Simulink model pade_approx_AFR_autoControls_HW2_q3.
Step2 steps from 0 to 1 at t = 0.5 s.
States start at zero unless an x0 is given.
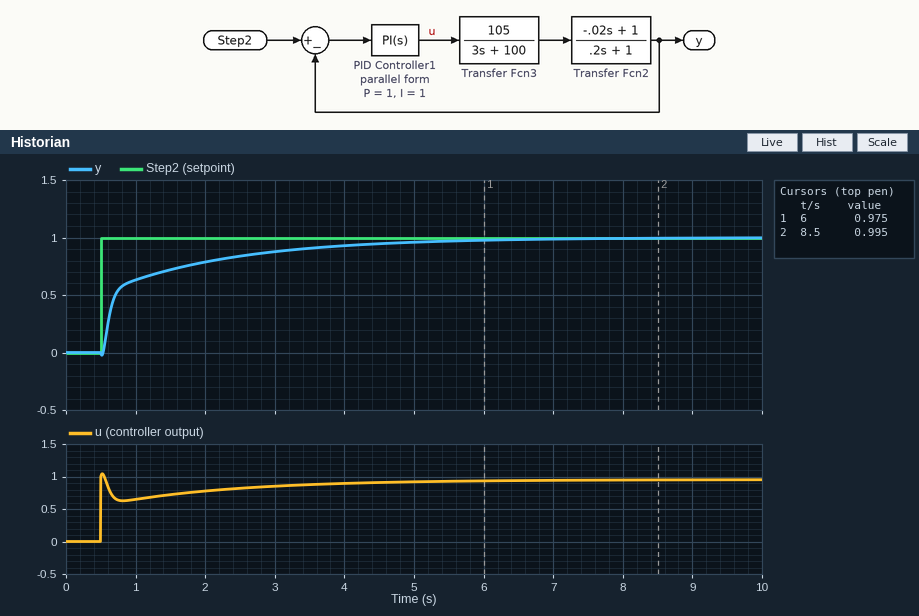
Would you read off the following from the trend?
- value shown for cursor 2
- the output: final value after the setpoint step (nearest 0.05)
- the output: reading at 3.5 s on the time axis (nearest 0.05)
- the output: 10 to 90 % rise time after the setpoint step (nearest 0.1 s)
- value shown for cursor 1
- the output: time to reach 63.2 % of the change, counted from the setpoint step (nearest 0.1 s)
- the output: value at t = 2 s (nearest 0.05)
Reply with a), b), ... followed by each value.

a) 0.995
b) 1.00
c) 0.90
d) 2.8 s
e) 0.975
f) 0.5 s
g) 0.80
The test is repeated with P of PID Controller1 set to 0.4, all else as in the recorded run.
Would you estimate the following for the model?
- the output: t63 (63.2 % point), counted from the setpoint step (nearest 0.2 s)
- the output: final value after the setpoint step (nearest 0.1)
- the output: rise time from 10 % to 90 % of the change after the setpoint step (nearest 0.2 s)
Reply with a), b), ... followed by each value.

a) 0.8 s
b) 1.0
c) 2.2 s
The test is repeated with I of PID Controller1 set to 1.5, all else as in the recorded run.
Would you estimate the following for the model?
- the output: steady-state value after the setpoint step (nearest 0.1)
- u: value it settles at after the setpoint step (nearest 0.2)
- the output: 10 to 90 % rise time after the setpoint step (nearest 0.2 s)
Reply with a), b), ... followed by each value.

a) 1.0
b) 1.0
c) 1.8 s
